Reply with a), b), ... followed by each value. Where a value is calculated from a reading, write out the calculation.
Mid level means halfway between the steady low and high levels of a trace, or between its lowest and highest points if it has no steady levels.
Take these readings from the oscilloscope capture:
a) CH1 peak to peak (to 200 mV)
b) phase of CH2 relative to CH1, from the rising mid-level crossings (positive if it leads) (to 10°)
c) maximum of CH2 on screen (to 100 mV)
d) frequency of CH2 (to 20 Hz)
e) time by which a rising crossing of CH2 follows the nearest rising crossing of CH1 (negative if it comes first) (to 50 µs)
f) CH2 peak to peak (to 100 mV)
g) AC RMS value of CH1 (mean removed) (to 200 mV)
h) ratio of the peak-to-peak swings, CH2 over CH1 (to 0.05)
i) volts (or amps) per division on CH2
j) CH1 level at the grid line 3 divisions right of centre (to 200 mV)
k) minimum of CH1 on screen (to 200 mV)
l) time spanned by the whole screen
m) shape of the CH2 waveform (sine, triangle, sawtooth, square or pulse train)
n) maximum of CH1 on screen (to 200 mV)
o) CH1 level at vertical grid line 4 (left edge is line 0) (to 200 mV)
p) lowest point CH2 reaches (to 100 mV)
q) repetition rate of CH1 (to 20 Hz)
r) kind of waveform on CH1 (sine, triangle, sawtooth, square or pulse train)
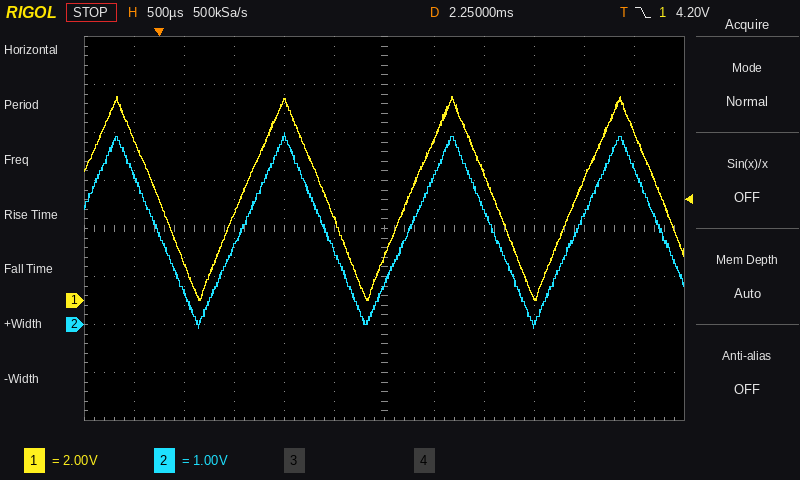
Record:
a) 8.4 V − (0.0 V) = 8.4 V
b) 0°
c) 4.0 V
d) 600 Hz
e) 0 µs
f) 4.0 V − (-100 mV) = 4.1 V
g) 8.4 V / (2√3) ≈ 2.4 V
h) 4.1 V / 8.4 V ≈ 0.488, so 0.50 to the nearest 0.05
i) 1 V
j) 200 mV
k) 0.0 V
l) 6 ms
m) triangle
n) 8.4 V
o) 8.2 V
p) -100 mV
q) 600 Hz
r) triangle
